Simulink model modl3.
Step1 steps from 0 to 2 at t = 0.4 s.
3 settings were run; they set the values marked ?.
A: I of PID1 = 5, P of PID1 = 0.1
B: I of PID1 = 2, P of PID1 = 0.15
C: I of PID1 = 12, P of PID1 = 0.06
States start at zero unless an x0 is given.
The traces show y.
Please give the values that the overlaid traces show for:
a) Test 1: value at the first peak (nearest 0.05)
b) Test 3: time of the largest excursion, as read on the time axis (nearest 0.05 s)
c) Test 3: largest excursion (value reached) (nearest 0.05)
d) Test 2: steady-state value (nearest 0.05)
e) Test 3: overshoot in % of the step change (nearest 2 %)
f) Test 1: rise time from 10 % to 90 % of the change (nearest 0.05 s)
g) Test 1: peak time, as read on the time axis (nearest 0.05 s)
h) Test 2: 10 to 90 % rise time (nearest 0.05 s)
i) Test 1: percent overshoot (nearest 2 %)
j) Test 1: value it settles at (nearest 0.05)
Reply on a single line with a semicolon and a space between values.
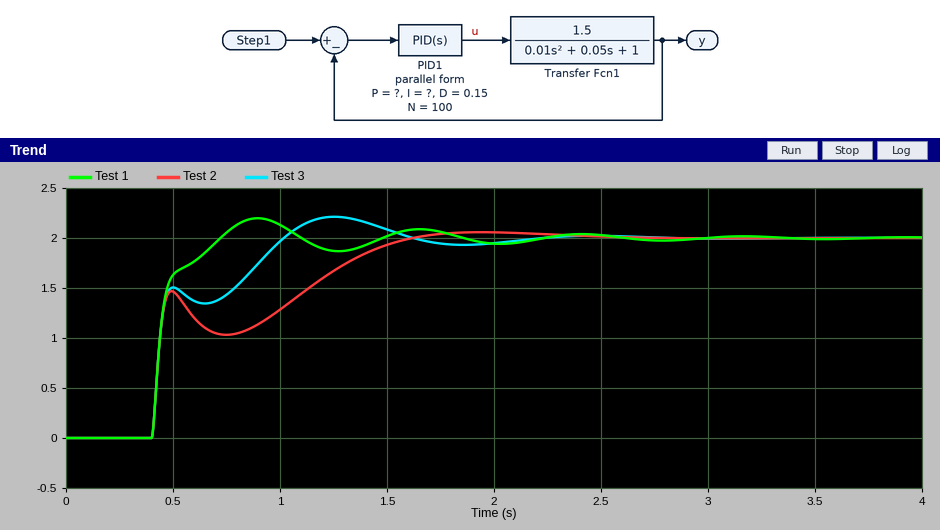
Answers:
2.20; 1.25 s; 2.20; 2.00; 10 %; 0.20 s; 0.90 s; 0.95 s; 10 %; 2.00
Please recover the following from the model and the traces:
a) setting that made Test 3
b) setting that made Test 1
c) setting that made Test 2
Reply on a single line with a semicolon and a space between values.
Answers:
A; C; B
